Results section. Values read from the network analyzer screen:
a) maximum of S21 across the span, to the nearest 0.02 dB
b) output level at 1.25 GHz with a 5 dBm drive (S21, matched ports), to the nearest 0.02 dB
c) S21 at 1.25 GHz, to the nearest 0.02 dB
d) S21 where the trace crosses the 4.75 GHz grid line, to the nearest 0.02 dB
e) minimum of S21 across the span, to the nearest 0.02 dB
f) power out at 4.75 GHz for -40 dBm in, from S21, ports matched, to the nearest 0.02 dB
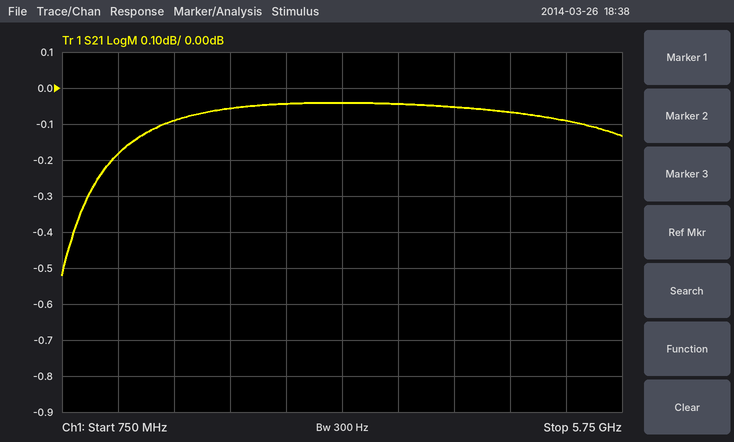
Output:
-0.04 dB
4.82 dBm
-0.18 dB
-0.06 dB
-0.52 dB
-40.06 dBm
